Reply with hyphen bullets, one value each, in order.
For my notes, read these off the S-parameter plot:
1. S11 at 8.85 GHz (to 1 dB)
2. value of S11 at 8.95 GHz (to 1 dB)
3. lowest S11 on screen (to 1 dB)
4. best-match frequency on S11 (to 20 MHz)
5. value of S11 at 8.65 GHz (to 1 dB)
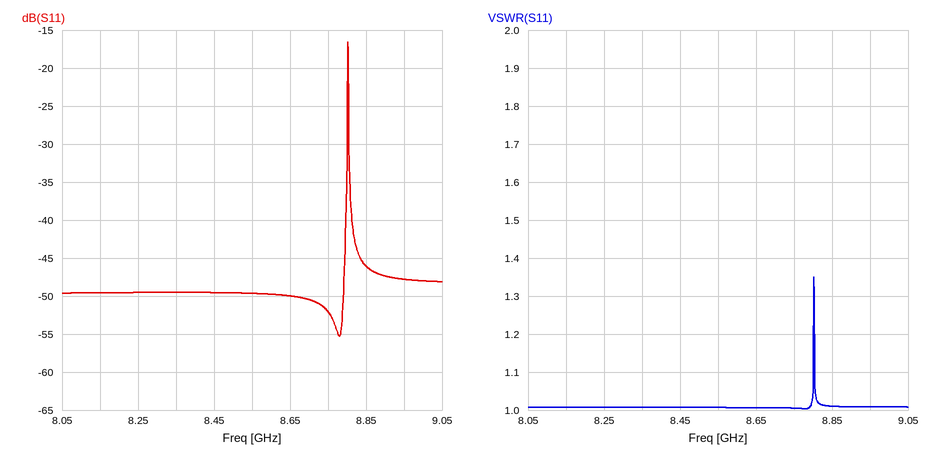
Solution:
- -46 dB
- -48 dB
- -55 dB
- 8.78 GHz
- -50 dB
